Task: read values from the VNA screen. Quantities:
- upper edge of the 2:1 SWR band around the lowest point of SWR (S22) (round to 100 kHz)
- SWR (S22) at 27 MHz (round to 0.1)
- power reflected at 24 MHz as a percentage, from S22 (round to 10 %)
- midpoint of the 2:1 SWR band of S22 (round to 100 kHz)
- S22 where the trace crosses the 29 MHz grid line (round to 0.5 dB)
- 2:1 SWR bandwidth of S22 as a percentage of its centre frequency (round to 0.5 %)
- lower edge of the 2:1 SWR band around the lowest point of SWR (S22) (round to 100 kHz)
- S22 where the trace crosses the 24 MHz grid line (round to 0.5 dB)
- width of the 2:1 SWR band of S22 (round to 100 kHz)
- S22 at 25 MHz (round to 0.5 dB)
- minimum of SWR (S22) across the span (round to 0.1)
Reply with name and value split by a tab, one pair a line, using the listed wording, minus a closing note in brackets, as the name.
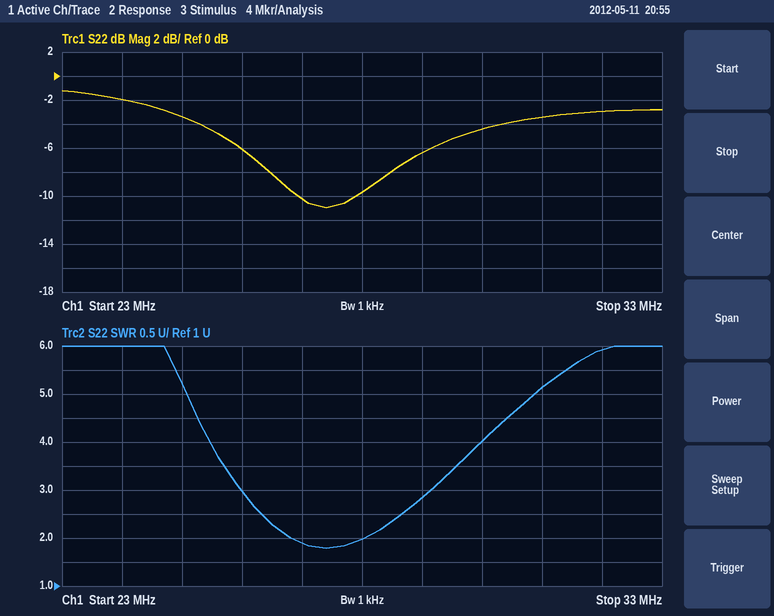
upper edge of the 2:1 SWR band around the lowest point of SWR (S22)	28.0 MHz
SWR (S22) at 27 MHz	1.9
power reflected at 24 MHz as a percentage, from S22	60 %
midpoint of the 2:1 SWR band of S22	27.4 MHz
S22 where the trace crosses the 29 MHz grid line	-6.5 dB
2:1 SWR bandwidth of S22 as a percentage of its centre frequency	4.5 %
lower edge of the 2:1 SWR band around the lowest point of SWR (S22)	26.8 MHz
S22 where the trace crosses the 24 MHz grid line	-2.0 dB
width of the 2:1 SWR band of S22	1.2 MHz
S22 at 25 MHz	-3.5 dB
minimum of SWR (S22) across the span	1.8
